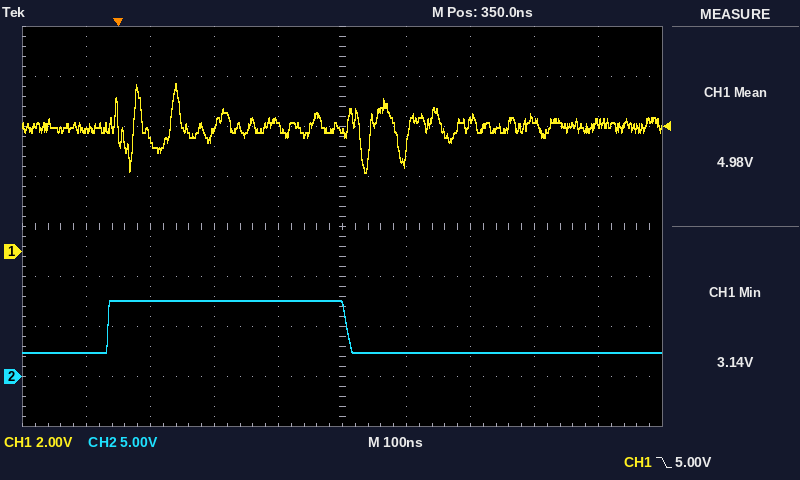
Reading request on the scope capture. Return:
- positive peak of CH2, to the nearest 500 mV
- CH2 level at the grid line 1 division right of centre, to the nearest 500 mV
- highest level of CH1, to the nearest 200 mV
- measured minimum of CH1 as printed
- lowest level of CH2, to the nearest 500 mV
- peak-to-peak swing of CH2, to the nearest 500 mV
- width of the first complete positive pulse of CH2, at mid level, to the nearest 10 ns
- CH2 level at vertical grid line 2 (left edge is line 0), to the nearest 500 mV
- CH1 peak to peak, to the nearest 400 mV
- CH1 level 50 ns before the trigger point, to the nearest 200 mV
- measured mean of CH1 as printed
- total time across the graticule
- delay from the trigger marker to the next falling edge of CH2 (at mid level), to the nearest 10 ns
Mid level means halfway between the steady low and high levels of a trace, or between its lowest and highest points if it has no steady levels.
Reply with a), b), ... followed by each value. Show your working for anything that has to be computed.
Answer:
a) 7.5 V
b) 2.5 V
c) 6.8 V
d) 3.14 V
e) 2.5 V
f) 7.5 V − (2.5 V) = 5.0 V
g) 370 ns
h) 7.5 V
i) 3.6 V
j) 4.8 V
k) 4.98 V
l) 1 µs
m) 360 ns
